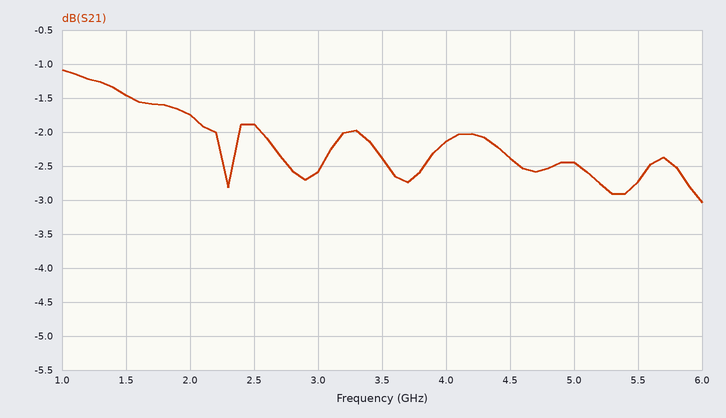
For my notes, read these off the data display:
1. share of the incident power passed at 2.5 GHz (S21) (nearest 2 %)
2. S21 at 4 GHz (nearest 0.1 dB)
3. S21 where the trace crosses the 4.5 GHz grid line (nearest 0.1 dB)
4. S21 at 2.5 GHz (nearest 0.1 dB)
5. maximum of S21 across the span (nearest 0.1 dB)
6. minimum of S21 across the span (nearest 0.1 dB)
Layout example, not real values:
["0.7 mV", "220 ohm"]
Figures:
["64 %", "-2.1 dB", "-2.4 dB", "-1.9 dB", "-1.1 dB", "-3.0 dB"]
